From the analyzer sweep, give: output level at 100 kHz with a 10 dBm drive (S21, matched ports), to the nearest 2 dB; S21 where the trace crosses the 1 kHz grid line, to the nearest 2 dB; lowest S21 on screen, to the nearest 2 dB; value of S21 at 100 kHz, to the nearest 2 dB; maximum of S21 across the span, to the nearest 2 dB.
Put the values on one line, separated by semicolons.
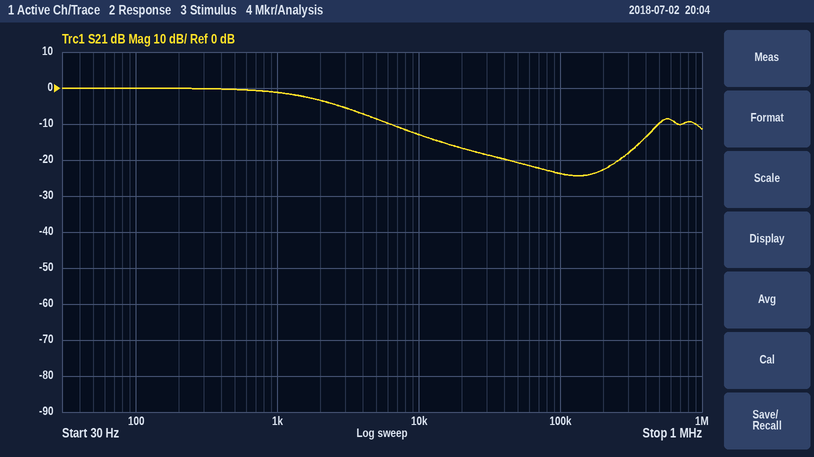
-14 dBm; -2 dB; -24 dB; -24 dB; 0 dB
